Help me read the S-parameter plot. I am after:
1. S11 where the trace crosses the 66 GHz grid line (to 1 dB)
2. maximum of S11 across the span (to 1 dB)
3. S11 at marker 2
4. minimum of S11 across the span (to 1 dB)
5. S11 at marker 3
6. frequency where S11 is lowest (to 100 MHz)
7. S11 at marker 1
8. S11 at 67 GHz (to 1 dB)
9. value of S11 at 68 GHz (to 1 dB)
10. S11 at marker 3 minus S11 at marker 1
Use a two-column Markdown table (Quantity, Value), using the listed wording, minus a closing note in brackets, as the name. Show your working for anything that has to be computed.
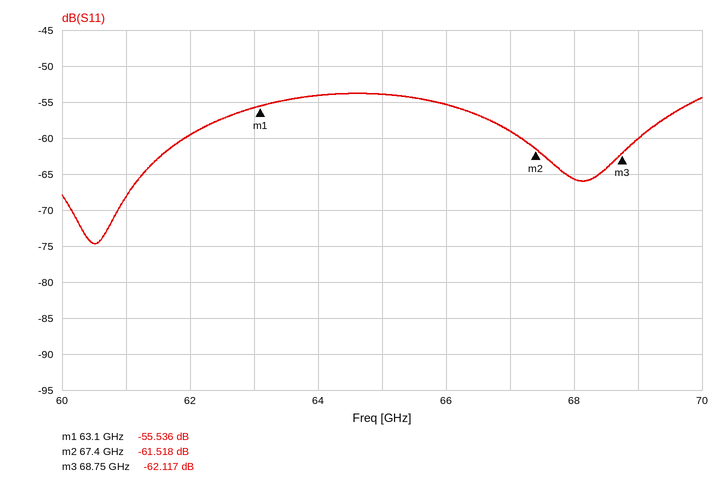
| Quantity | Value |
|---|---|
| S11 where the trace crosses the 66 GHz grid line | -55 dB |
| maximum of S11 across the span | -54 dB |
| S11 at marker 2 | -61.518 dB |
| minimum of S11 across the span | -75 dB |
| S11 at marker 3 | -62.117 dB |
| frequency where S11 is lowest | 60.5 GHz |
| S11 at marker 1 | -55.536 dB |
| S11 at 67 GHz | -59 dB |
| value of S11 at 68 GHz | -66 dB |
| S11 at marker 3 minus S11 at marker 1 | -62.117 − (-55.536) = -6.581 dB |
